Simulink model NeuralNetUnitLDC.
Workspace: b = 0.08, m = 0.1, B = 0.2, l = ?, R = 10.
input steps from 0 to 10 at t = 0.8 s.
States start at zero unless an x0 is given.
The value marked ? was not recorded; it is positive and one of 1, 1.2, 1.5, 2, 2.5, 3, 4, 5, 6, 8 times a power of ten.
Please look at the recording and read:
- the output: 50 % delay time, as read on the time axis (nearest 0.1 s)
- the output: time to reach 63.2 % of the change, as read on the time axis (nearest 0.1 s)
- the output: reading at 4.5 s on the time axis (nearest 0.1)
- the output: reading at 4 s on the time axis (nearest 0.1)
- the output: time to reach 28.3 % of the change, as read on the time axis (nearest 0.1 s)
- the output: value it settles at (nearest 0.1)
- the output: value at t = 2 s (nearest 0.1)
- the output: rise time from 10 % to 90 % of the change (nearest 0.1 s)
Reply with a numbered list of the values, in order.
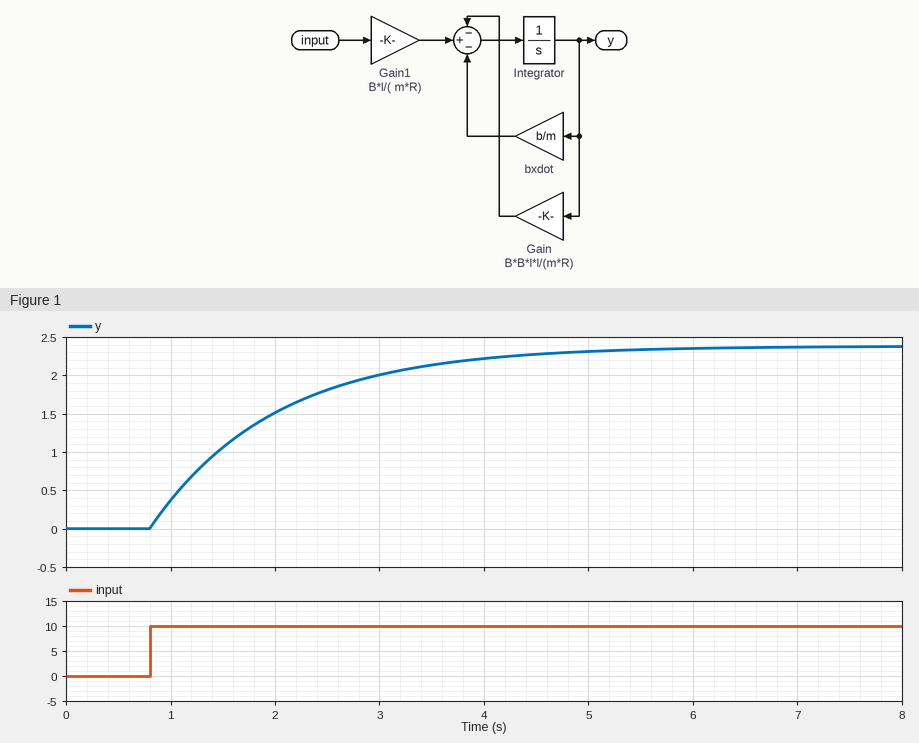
1. 1.6 s
2. 2.0 s
3. 2.3
4. 2.2
5. 1.2 s
6. 2.4
7. 1.5
8. 2.6 s
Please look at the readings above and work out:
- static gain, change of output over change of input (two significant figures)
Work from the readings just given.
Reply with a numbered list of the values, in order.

1. 0.24
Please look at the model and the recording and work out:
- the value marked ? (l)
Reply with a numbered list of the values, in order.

1. 1
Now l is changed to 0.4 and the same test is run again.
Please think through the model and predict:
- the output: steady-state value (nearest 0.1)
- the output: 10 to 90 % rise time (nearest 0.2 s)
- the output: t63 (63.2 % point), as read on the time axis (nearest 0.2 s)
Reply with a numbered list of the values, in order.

1. 1.0
2. 2.8 s
3. 2.0 s
